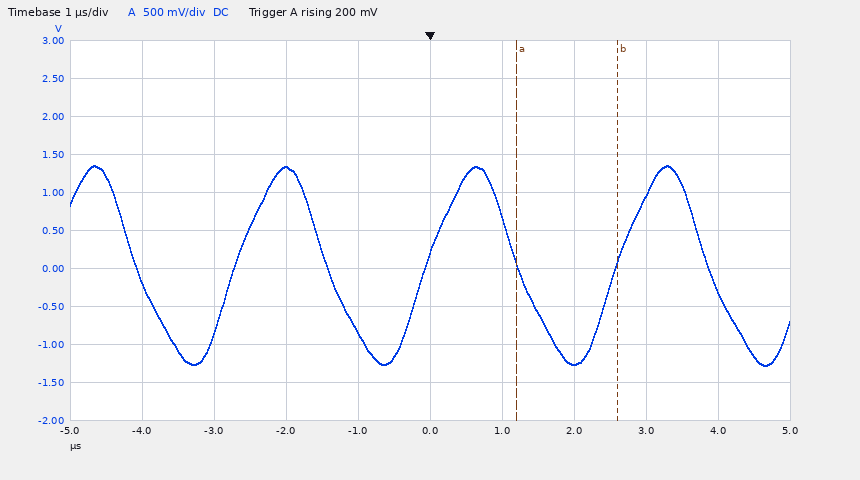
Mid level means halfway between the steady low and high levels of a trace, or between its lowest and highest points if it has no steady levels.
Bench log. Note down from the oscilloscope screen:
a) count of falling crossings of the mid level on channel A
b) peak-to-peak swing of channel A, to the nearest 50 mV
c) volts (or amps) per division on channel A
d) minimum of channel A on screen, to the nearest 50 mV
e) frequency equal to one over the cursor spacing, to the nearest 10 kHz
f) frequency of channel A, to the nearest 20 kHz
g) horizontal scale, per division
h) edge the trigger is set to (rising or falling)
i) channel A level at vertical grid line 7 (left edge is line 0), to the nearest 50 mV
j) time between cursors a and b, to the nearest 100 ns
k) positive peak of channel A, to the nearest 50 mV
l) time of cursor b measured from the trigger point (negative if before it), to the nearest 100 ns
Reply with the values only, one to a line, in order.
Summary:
4
2.65 V
500 mV
-1.30 V
710 kHz
380 kHz
1 µs
rising
-1.25 V
1.4 µs
1.35 V
+2.6 µs
